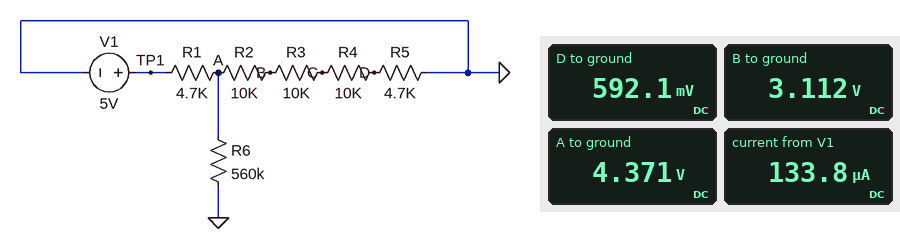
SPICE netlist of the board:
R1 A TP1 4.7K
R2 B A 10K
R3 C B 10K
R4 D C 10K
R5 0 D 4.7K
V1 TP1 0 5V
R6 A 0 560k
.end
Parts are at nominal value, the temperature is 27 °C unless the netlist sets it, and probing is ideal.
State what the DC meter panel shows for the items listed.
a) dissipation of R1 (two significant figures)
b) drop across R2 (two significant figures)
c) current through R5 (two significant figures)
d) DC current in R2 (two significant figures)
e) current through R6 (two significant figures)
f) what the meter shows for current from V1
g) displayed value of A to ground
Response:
84 µW
1.3 V
130 µA
130 µA
7.8 µA
133.8 µA
4.371 V
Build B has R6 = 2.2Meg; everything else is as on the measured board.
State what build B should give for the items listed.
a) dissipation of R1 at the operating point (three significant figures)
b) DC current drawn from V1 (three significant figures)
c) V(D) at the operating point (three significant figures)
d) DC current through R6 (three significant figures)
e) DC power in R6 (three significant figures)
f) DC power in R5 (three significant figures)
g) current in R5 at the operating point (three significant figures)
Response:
77.8 µW
129 µA
595 mV
2.00 µA
8.78 µW
75.4 µW
127 µA
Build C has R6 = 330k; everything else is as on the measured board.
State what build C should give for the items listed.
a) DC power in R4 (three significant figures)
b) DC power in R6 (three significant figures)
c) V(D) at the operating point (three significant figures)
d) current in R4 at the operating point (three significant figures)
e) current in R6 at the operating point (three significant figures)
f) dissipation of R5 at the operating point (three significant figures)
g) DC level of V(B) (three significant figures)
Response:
157 µW
57.3 µW
589 mV
125 µA
13.2 µA
73.8 µW
3.10 V
